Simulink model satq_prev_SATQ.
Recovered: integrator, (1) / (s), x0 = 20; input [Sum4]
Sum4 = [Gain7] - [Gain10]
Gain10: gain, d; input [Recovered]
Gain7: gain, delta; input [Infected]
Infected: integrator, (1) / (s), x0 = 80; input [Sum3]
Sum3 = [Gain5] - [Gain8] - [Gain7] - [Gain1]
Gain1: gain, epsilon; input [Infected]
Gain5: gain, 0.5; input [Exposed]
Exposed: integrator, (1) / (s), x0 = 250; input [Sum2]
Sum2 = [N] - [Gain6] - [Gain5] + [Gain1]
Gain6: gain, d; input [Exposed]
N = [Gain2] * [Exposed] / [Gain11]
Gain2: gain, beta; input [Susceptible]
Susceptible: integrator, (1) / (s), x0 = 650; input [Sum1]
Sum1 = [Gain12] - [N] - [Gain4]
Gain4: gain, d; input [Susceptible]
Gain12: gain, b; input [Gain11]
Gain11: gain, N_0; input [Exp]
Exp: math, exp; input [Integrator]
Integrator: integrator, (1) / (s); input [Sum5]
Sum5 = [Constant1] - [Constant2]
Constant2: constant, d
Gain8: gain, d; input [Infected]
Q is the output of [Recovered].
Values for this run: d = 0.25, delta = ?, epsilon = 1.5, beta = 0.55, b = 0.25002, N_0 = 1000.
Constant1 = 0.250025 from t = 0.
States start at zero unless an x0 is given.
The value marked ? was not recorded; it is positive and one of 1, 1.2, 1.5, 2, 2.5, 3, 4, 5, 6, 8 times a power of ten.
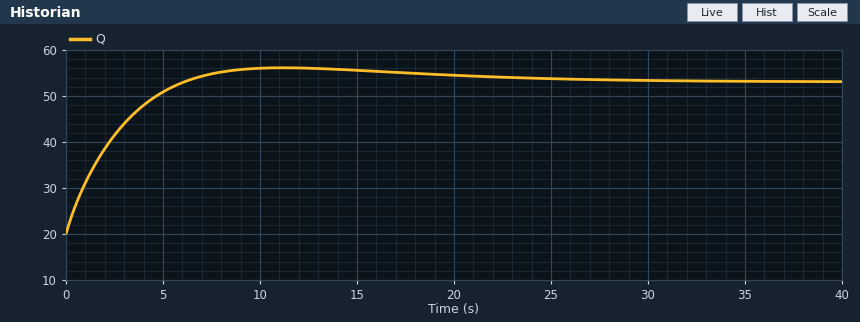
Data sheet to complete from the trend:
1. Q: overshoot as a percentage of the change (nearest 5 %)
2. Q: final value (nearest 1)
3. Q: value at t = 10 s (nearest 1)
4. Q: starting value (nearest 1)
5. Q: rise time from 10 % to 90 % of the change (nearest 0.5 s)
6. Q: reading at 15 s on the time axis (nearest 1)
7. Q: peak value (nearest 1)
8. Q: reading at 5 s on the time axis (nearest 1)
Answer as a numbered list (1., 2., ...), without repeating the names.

1. 10 %
2. 53
3. 56
4. 20
5. 4.5 s
6. 56
7. 56
8. 51
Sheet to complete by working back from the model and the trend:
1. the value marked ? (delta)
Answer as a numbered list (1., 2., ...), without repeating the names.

1. 0.25
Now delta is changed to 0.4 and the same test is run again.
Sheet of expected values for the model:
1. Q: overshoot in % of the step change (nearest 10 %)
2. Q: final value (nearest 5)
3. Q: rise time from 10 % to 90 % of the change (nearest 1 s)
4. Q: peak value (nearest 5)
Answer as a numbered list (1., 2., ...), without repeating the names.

1. 30 %
2. 65
3. 3 s
4. 75
